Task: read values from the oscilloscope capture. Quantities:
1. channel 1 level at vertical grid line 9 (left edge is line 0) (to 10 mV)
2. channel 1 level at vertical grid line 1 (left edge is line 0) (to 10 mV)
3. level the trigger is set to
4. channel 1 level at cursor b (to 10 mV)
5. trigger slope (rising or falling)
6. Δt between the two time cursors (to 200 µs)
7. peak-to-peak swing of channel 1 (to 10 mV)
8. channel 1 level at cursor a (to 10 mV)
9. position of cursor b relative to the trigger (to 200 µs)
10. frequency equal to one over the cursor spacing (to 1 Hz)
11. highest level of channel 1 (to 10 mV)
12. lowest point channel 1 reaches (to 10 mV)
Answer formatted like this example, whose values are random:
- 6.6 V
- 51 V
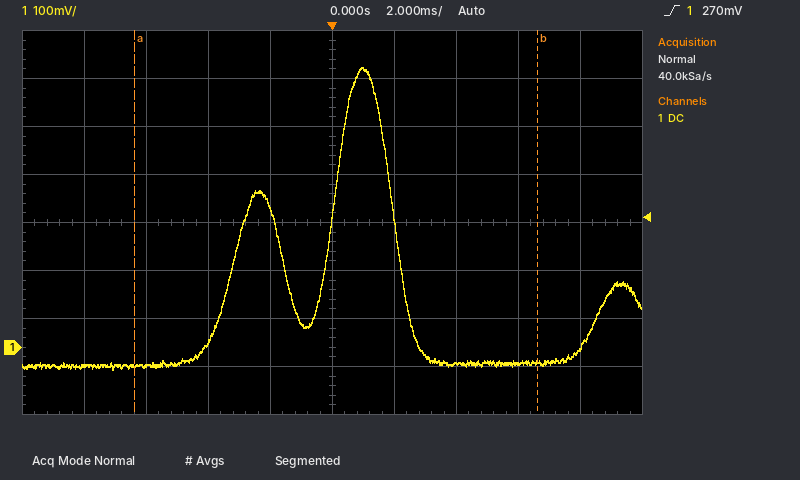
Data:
- 0 mV
- -40 mV
- 270 mV
- -30 mV
- rising
- 13.0 ms
- 630 mV
- -40 mV
- +6.6 ms
- 77 Hz
- 580 mV
- -50 mV
